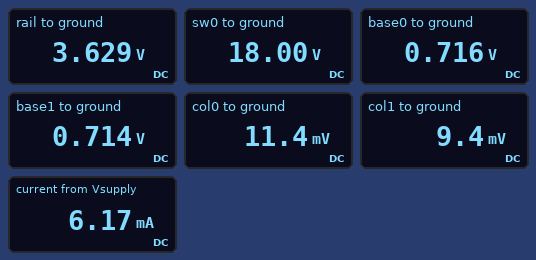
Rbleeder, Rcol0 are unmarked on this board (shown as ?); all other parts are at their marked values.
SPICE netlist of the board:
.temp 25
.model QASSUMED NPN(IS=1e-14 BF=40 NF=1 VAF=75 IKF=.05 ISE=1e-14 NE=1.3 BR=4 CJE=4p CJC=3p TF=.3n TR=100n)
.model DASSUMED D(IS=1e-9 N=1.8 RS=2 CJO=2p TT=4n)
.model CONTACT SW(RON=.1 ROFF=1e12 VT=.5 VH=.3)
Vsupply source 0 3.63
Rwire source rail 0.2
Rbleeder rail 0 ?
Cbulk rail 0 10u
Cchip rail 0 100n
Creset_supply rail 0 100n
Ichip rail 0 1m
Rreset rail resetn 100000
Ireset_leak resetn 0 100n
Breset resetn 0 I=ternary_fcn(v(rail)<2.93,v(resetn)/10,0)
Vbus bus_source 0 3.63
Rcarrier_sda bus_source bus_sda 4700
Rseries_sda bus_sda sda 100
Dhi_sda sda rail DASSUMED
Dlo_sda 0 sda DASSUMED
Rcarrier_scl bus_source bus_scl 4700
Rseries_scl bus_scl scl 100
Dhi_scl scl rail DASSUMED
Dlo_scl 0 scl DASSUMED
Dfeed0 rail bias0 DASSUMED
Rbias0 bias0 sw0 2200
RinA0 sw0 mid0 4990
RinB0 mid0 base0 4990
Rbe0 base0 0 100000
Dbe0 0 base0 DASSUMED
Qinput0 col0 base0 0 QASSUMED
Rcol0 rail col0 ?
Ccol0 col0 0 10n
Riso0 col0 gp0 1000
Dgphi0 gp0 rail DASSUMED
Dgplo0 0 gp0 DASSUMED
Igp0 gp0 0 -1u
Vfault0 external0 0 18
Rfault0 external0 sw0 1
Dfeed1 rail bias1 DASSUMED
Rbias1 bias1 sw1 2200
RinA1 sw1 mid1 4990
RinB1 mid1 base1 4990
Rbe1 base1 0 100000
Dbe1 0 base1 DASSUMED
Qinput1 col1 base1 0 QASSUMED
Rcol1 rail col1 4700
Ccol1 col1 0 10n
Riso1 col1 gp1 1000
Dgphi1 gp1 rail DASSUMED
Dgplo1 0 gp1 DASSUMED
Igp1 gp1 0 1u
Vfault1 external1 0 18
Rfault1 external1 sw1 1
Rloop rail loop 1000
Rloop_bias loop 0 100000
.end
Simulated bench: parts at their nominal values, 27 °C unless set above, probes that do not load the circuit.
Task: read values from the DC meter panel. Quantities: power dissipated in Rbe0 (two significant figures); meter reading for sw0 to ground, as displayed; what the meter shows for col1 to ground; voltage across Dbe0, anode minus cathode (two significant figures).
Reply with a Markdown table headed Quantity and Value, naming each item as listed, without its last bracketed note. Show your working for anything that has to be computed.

| Quantity | Value |
|---|---|
| power dissipated in Rbe0 | (716 mV)^2 / 100 kΩ = 5.1 µW |
| meter reading for sw0 to ground, as displayed | 18.00 V |
| what the meter shows for col1 to ground | 9.4 mV |
| voltage across Dbe0, anode minus cathode | 0 V - 716 mV = -720 mV |
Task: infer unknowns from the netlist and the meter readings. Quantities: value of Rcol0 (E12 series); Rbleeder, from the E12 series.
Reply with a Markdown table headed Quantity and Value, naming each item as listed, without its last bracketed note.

| Quantity | Value |
|---|---|
| value of Rcol0 | 2.7 kΩ |
| Rbleeder, from the E12 series | 1.2 kΩ |
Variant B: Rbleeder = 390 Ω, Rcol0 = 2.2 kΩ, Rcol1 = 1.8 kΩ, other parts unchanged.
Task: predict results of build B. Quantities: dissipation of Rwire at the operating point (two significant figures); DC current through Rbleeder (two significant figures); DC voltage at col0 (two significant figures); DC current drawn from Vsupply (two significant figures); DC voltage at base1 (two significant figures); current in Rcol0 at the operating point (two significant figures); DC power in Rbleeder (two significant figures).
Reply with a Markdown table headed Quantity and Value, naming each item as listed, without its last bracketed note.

| Quantity | Value |
|---|---|
| dissipation of Rwire at the operating point | 39 µW |
| DC current through Rbleeder | 9.3 mA |
| DC voltage at col0 | 12 mV |
| DC current drawn from Vsupply | 14 mA |
| DC voltage at base1 | 720 mV |
| current in Rcol0 at the operating point | 1.6 mA |
| DC power in Rbleeder | 34 mW |
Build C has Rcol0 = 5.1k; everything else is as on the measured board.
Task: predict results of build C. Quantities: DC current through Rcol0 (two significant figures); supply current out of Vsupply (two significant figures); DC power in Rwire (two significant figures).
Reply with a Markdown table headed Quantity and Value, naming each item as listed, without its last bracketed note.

| Quantity | Value |
|---|---|
| DC current through Rcol0 | 710 µA |
| supply current out of Vsupply | 5.5 mA |
| DC power in Rwire | 6.1 µW |
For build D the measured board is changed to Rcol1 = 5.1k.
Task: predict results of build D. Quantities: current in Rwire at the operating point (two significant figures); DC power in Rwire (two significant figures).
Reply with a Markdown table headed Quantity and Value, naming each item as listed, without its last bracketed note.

| Quantity | Value |
|---|---|
| current in Rwire at the operating point | 6.1 mA |
| DC power in Rwire | 7.5 µW |
